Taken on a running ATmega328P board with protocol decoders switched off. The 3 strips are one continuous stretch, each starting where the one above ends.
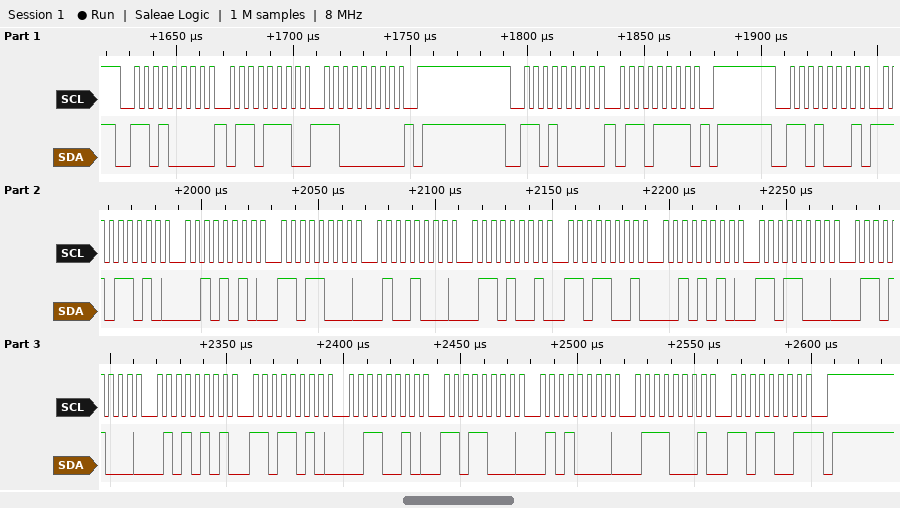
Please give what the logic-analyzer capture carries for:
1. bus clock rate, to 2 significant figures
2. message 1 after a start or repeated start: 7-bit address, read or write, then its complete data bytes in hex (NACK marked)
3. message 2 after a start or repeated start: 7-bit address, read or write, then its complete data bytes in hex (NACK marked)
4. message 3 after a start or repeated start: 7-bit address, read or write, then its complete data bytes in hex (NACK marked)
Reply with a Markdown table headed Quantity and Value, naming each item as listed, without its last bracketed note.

| Quantity | Value |
|---|---|
| bus clock rate, to 2 significant figures | 250 kHz |
| message 1 after a start or repeated start: 7-bit address, read or write, then its complete data bytes in hex | 0x68 write: 6E C0 |
| message 2 after a start or repeated start: 7-bit address, read or write, then its complete data bytes in hex | 0x68 write: 6F |
| message 3 after a start or repeated start: 7-bit address, read or write, then its complete data bytes in hex | 0x68 read: DA 2A D8 48 69 D9 2A D8 68 55 DA 32 D8 50 71 D9 NACK |
